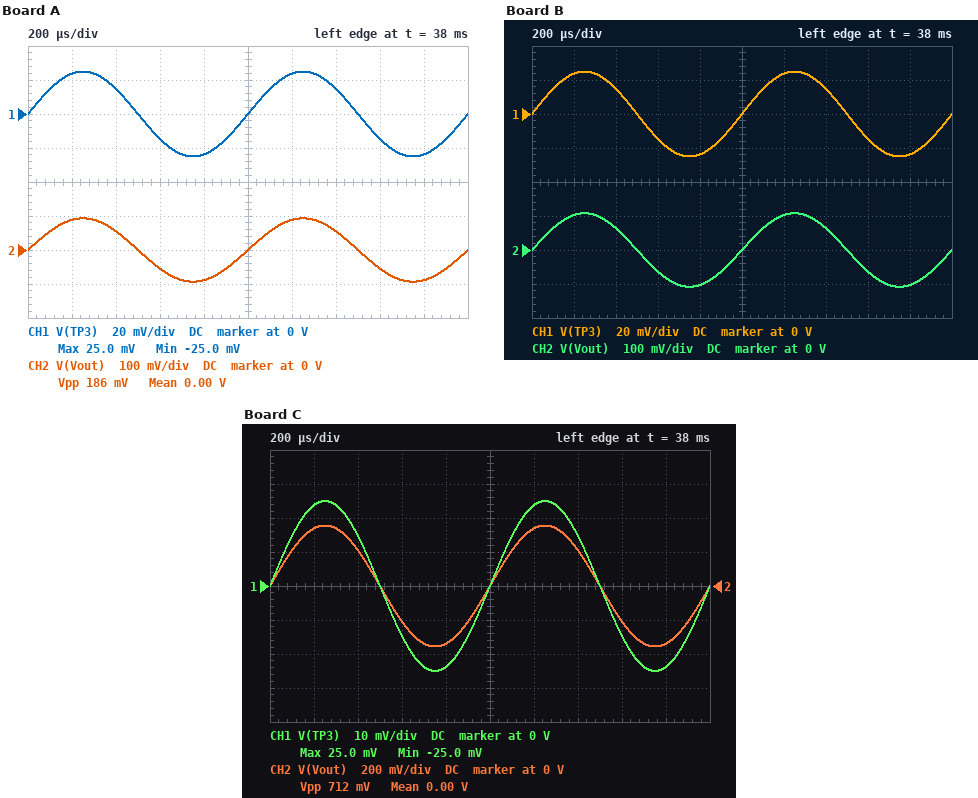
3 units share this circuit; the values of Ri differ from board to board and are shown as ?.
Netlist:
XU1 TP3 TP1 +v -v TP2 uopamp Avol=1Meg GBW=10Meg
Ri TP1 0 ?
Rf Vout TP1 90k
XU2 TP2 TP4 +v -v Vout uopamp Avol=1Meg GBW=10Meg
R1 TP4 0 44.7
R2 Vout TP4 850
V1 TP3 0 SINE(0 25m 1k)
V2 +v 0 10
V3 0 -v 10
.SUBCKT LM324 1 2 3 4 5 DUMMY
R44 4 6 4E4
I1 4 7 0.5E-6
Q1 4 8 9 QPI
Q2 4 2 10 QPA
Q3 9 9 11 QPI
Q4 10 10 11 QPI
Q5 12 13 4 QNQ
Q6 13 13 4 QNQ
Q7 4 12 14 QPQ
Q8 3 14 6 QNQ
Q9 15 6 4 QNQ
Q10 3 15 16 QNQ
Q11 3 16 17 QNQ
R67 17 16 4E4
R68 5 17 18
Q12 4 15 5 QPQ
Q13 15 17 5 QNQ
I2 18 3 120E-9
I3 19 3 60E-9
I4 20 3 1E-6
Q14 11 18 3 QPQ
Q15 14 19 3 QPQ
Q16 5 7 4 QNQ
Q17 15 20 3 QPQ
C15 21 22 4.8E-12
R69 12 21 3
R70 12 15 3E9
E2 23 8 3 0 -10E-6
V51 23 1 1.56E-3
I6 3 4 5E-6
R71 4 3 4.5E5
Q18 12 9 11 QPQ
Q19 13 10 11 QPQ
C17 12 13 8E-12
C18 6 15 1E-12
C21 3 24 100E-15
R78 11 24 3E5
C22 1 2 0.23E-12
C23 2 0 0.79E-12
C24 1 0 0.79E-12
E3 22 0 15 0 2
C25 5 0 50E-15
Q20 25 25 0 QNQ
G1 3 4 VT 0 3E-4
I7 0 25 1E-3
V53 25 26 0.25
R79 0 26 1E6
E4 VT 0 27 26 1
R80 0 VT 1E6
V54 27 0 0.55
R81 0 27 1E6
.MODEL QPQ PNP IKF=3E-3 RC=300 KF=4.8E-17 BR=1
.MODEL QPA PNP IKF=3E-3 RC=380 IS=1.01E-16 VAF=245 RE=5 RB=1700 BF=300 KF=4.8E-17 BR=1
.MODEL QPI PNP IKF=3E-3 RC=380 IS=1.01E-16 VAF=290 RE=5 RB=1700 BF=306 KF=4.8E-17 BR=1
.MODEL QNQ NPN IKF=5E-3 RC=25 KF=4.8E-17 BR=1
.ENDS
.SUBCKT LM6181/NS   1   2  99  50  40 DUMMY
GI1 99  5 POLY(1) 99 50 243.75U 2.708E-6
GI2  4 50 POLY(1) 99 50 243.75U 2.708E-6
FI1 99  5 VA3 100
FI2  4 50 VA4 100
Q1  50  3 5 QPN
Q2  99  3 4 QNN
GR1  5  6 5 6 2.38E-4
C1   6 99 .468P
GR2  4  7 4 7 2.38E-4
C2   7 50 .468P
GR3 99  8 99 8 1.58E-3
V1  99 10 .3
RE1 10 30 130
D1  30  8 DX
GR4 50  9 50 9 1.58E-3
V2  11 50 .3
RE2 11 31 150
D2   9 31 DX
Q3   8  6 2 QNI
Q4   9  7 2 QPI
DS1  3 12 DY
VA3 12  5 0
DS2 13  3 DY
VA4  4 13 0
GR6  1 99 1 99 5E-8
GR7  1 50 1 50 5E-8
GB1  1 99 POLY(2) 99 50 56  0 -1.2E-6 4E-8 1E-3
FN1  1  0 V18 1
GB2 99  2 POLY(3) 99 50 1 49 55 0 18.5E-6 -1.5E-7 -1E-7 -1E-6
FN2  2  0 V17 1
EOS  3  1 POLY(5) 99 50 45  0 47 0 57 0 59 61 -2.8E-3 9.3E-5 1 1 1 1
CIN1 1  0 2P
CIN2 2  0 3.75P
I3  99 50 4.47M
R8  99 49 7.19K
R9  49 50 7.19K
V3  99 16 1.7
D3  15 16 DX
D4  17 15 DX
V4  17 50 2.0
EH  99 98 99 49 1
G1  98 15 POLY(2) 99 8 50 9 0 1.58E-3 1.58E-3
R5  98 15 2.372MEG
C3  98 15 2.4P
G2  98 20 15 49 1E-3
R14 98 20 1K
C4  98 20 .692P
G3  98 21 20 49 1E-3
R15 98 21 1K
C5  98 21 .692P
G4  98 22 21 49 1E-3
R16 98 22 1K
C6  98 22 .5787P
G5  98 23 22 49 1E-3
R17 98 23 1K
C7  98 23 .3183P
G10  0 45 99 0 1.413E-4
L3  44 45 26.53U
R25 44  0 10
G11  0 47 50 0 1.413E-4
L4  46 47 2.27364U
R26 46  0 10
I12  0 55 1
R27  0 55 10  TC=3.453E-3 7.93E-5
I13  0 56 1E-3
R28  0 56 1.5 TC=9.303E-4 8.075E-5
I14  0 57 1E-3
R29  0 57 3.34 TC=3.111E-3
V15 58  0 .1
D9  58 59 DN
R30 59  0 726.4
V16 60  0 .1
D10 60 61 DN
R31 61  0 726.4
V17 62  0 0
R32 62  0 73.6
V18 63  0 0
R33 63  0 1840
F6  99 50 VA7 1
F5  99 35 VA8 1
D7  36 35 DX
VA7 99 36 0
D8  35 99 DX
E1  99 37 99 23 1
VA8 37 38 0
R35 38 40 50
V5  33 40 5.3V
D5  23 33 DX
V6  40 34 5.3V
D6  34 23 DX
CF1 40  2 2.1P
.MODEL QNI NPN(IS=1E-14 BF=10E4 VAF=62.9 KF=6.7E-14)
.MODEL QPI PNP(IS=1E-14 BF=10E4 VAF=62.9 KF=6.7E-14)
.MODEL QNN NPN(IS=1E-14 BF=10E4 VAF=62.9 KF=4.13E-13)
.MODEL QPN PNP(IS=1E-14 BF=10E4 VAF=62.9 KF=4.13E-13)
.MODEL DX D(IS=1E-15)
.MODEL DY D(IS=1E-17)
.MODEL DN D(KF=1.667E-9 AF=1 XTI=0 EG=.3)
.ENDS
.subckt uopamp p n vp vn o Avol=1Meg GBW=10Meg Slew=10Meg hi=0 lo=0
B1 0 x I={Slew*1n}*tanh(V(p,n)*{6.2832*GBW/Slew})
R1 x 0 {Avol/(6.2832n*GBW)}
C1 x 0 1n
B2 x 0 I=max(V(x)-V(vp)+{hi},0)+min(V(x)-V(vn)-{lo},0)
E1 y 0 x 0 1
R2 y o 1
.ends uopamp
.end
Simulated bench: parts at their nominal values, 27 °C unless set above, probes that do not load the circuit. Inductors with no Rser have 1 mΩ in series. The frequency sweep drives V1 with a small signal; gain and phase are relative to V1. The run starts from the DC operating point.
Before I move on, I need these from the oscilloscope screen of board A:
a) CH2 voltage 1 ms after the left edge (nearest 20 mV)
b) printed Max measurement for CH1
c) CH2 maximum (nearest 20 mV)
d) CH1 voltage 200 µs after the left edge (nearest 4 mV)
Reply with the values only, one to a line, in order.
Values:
0 V
25.0 mV
100 mV
24 mV
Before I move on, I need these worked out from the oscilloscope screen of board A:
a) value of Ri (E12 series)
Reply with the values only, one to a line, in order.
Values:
33 kΩ
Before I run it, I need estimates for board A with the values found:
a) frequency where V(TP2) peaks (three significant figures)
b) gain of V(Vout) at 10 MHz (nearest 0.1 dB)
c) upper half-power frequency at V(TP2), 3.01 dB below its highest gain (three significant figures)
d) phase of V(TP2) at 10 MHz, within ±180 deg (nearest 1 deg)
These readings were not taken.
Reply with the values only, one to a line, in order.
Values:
5.18 MHz
2.7 dB
5.43 MHz
-89 deg
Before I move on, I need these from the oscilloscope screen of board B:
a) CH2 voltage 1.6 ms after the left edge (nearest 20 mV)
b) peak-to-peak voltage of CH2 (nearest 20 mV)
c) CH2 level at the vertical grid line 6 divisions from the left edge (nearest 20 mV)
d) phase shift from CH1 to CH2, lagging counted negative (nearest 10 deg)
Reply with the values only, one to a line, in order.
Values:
-60 mV
220 mV
100 mV
0 deg
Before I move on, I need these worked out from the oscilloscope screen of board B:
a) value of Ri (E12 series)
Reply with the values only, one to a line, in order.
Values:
27 kΩ
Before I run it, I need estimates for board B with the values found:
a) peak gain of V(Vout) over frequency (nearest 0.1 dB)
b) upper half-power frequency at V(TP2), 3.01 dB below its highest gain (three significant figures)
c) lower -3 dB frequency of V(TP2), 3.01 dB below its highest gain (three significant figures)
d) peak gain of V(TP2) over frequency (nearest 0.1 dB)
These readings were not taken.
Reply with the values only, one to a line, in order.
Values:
32.4 dB
5.06 MHz
4.56 MHz
26.1 dB
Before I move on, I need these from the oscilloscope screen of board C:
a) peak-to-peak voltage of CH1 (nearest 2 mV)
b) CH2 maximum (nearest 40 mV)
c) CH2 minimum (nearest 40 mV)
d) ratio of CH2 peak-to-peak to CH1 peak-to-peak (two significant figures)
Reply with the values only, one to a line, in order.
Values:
50 mV
360 mV
-360 mV
14
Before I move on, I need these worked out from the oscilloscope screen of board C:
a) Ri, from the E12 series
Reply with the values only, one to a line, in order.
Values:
6.8 kΩ
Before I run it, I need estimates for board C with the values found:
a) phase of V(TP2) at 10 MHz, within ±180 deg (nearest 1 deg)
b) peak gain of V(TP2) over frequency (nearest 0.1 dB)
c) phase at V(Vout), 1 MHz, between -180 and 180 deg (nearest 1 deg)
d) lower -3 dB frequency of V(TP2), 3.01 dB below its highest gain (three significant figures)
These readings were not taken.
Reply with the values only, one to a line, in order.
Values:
-90 deg
26.2 dB
-5 deg
2.41 MHz
